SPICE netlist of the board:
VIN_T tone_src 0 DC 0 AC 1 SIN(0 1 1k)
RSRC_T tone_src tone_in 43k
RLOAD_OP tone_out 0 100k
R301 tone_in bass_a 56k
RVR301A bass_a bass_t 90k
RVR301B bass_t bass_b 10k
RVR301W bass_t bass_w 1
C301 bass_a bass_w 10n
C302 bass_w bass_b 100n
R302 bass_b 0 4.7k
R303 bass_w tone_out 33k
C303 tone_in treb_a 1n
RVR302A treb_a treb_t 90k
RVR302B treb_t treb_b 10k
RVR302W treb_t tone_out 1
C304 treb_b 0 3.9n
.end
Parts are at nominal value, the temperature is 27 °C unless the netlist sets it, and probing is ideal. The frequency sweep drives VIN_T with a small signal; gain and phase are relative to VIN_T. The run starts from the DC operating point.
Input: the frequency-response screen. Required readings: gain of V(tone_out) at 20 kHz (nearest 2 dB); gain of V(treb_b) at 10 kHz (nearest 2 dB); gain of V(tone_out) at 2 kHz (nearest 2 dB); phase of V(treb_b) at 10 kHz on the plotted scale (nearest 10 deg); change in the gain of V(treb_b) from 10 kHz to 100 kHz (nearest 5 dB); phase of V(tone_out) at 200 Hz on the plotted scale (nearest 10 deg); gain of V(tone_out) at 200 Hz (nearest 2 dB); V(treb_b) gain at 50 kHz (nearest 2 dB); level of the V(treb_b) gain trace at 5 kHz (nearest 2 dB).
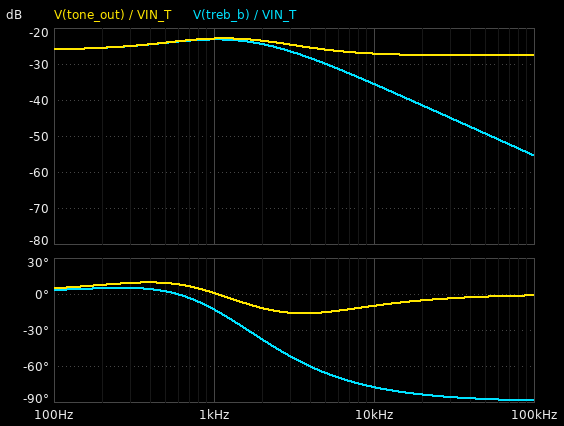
-28 dB
-36 dB
-24 dB
-80 deg
-20 dB
10 deg
-26 dB
-50 dB
-30 dB
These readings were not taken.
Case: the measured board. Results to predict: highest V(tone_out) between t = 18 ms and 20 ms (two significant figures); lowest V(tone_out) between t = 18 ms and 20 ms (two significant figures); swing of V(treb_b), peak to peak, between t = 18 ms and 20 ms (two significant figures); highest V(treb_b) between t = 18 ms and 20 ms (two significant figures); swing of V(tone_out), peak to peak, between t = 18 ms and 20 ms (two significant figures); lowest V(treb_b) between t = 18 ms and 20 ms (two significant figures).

71 mV
-71 mV
140 mV
69 mV
140 mV
-69 mV
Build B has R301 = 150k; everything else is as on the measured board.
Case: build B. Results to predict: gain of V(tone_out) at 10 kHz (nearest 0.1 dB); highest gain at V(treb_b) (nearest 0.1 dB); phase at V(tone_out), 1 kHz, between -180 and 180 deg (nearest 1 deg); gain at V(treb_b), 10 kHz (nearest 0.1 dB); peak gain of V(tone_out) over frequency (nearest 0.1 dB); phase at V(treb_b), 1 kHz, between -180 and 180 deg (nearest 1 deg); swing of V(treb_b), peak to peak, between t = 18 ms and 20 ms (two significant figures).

-26.0 dB
-22.3 dB
11 deg
-34.5 dB
-21.9 dB
-3 deg
150 mV
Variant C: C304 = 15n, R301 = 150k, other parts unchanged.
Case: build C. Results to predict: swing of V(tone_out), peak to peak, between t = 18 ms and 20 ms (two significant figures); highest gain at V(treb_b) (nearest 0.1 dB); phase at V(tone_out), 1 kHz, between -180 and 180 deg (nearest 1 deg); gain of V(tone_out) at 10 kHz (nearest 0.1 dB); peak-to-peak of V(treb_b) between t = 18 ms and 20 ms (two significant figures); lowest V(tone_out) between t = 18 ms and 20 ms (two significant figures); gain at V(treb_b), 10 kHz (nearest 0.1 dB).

81 mV
-29.5 dB
11 deg
-26.6 dB
59 mV
-41 mV
-46.1 dB
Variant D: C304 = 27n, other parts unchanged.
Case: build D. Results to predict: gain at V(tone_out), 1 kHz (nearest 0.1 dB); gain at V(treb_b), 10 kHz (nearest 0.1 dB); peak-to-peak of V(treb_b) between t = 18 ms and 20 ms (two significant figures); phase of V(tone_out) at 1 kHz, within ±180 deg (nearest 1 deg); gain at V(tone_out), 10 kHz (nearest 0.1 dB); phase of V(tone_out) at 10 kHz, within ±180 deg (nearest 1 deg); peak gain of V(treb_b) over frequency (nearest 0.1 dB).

-30.3 dB
-52.3 dB
31 mV
10 deg
-27.7 dB
3 deg
-26.2 dB
